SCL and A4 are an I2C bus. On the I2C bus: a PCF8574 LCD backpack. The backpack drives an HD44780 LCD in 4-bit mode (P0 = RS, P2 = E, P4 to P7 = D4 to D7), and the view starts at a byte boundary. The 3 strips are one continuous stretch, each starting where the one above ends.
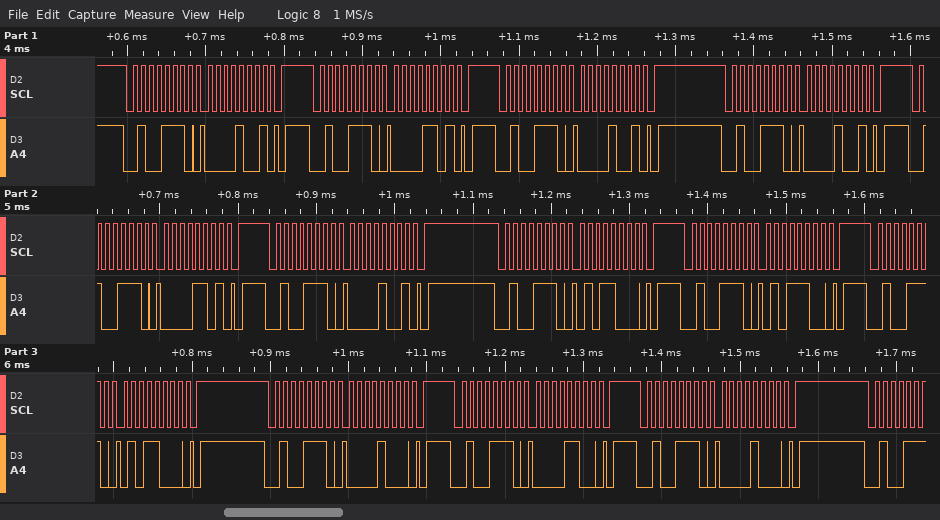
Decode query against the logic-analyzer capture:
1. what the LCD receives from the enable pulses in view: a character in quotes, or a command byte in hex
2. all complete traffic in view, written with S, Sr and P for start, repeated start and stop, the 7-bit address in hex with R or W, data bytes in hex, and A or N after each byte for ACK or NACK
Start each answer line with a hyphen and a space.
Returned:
- data 0x00 0x50
- S 27W A 09 A P S 27W A 0D A P S 27W A 09 A P S 27W A 09 A P S 27W A 0D A P S 27W A 09 A P S 27W A 58 A P S 27W A 5C A P S 27W A 58 A P S 27W A 08 A P S 27W A 0C A P S 27W A 08 A P
